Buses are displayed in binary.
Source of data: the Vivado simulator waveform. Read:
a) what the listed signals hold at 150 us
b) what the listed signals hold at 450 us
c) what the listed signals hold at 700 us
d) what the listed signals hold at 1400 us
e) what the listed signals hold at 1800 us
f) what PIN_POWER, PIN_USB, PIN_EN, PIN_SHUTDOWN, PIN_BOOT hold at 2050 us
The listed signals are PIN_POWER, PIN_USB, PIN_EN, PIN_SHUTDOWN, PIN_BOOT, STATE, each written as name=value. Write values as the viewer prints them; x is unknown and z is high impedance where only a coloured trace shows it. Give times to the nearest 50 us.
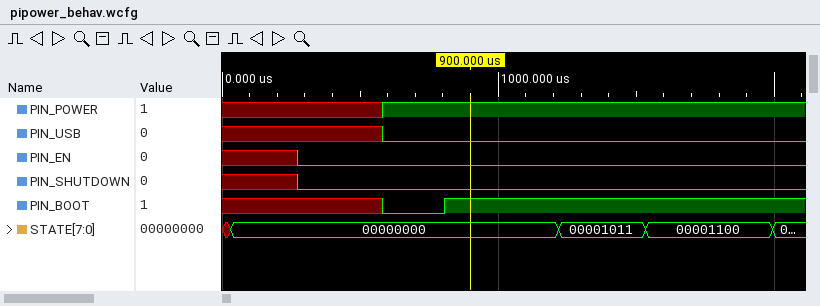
PIN_POWER=x, PIN_USB=x, PIN_EN=x, PIN_SHUTDOWN=x, PIN_BOOT=x, STATE=00000000
PIN_POWER=x, PIN_USB=x, PIN_EN=0, PIN_SHUTDOWN=0, PIN_BOOT=x, STATE=00000000
PIN_POWER=1, PIN_USB=0, PIN_EN=0, PIN_SHUTDOWN=0, PIN_BOOT=0, STATE=00000000
PIN_POWER=1, PIN_USB=0, PIN_EN=0, PIN_SHUTDOWN=0, PIN_BOOT=1, STATE=00001011
PIN_POWER=1, PIN_USB=0, PIN_EN=0, PIN_SHUTDOWN=0, PIN_BOOT=1, STATE=00001100
PIN_POWER=1, PIN_USB=0, PIN_EN=0, PIN_SHUTDOWN=0, PIN_BOOT=1
